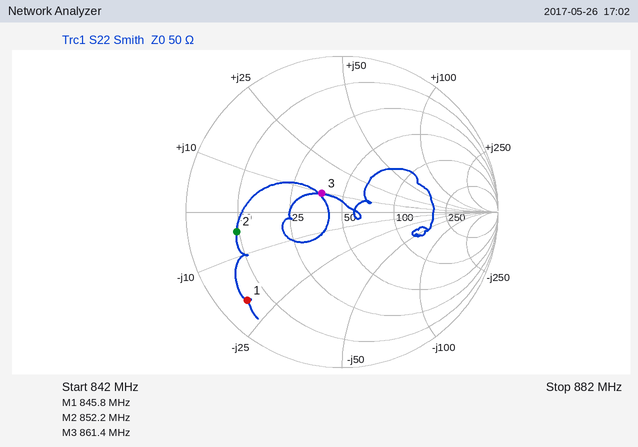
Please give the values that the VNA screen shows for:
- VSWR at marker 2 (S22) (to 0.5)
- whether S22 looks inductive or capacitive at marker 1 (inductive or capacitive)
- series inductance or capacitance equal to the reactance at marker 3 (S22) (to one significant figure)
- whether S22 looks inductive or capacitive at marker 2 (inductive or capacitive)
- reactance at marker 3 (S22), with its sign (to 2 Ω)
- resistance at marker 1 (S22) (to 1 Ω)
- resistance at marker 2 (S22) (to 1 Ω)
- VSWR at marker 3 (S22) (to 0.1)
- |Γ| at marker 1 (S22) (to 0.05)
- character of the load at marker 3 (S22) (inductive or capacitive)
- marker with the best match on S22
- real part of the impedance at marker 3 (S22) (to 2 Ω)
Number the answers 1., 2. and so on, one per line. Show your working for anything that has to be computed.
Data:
1. 5.5
2. capacitive
3. L = 10 Ω/(2π × 861.4 MHz) ≈ 2 nH
4. capacitive
5. +10 Ω
6. 5 Ω
7. 9 Ω
8. 1.4
9. 0.85
10. inductive
11. marker 3
12. 38 Ω
